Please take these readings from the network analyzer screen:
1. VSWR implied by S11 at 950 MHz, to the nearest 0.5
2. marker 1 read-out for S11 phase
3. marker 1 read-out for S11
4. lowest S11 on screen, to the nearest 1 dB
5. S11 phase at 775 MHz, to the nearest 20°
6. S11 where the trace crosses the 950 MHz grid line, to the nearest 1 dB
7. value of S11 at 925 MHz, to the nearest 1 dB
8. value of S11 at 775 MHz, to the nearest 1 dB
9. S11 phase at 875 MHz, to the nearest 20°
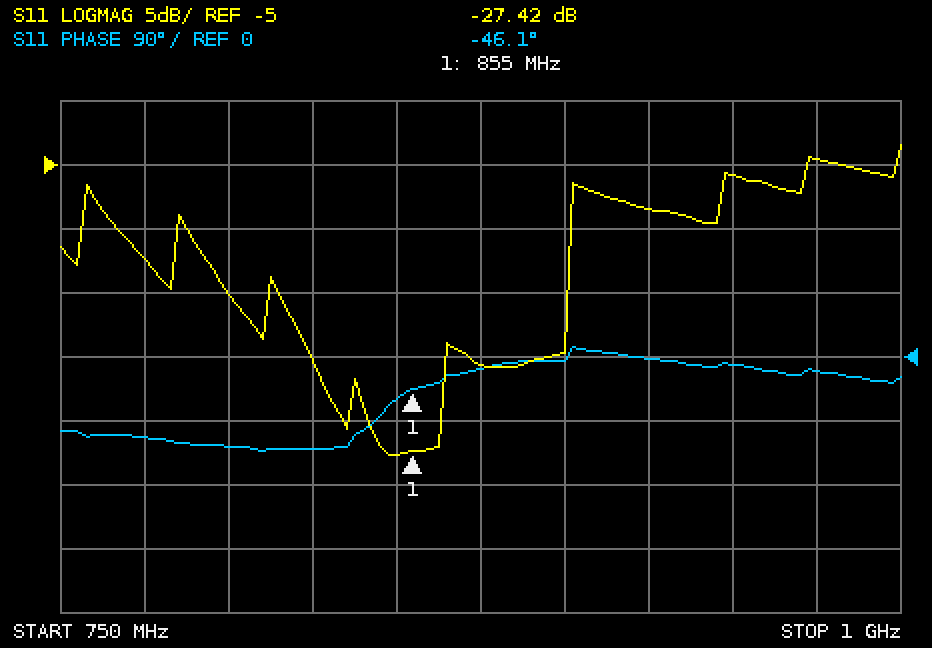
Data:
3.0
-46.1°
-27.42 dB
-28 dB
-120°
-6 dB
-8 dB
-12 dB
-20°
